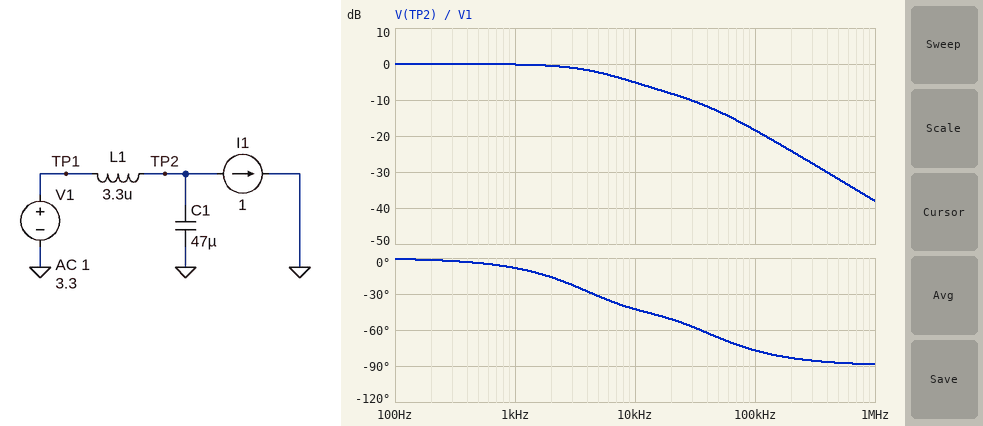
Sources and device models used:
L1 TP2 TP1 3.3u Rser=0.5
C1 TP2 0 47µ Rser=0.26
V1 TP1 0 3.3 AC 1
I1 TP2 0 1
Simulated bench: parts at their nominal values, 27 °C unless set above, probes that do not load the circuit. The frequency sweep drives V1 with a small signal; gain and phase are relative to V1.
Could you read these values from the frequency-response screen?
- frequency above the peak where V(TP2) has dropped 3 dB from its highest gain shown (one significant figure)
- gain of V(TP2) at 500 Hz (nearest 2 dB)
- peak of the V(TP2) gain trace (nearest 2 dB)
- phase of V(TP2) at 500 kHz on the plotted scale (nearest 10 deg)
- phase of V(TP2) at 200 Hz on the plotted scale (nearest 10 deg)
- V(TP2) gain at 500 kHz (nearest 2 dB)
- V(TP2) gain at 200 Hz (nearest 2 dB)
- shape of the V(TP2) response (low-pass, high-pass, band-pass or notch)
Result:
6 kHz
0 dB
0 dB
-90 deg
0 deg
-32 dB
0 dB
low-pass
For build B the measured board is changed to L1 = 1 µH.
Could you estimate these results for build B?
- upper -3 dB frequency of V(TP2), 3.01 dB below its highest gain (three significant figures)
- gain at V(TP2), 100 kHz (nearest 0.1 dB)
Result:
5.35 kHz
-11.3 dB
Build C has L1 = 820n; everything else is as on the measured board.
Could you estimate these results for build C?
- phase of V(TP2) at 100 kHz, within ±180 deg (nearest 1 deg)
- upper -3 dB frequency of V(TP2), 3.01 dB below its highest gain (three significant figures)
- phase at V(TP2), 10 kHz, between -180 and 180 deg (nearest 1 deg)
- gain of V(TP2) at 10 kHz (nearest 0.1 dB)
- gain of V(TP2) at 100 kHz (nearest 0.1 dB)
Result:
-40 deg
5.30 kHz
-32 deg
-5.6 dB
-10.7 dB
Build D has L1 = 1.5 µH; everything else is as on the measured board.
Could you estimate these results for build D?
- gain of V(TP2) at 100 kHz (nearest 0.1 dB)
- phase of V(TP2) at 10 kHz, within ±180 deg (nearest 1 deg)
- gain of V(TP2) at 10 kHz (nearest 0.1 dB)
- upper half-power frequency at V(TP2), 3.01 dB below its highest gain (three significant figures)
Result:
-13.1 dB
-35 deg
-5.4 dB
5.48 kHz
